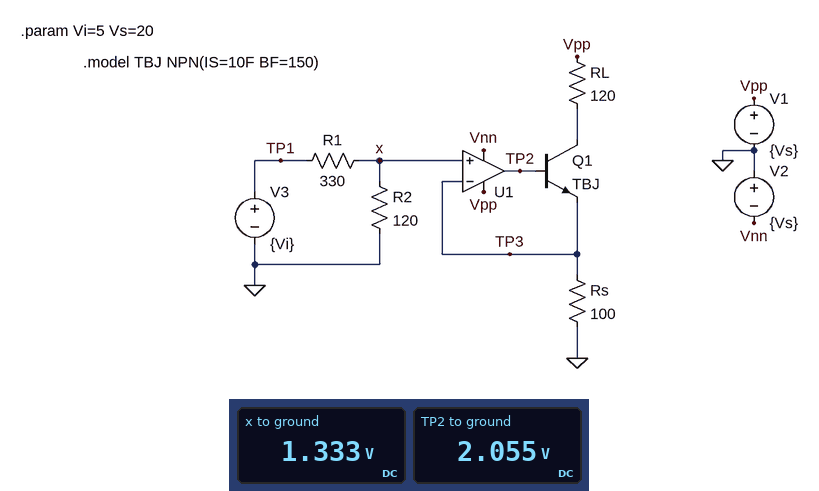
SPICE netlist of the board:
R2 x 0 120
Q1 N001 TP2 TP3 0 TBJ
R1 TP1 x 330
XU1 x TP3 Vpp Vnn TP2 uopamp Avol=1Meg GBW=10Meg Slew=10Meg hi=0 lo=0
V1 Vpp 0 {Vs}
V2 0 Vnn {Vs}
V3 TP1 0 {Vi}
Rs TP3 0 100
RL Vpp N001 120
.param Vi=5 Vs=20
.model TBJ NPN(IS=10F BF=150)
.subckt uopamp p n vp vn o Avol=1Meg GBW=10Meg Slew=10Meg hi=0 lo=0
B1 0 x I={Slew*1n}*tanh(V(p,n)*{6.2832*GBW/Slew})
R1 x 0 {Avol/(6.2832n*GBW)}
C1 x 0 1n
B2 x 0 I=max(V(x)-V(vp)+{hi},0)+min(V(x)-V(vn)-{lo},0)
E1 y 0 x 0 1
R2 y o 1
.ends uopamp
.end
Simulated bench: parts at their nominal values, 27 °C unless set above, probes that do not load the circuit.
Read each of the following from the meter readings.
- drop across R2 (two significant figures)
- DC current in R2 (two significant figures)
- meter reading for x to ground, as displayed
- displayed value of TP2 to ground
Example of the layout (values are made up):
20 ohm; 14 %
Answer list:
1.3 V; 11 mA; 1.333 V; 2.055 V
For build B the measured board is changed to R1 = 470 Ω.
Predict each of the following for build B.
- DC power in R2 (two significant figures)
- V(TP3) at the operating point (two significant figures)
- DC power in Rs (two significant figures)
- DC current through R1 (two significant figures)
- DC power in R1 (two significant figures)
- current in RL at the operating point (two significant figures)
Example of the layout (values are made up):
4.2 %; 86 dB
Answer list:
8.6 mW; 1.0 V; 10 mW; 8.5 mA; 34 mW; 10 mA
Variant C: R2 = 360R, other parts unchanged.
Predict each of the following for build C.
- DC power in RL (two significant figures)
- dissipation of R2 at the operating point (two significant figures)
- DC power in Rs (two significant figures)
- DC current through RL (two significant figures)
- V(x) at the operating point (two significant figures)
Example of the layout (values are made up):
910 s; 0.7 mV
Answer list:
81 mW; 19 mW; 68 mW; 26 mA; 2.6 V
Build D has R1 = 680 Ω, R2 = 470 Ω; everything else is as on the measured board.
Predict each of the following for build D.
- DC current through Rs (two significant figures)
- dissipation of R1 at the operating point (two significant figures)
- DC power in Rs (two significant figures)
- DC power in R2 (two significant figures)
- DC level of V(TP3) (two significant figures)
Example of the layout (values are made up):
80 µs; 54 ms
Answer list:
20 mA; 13 mW; 42 mW; 8.9 mW; 2.0 V
